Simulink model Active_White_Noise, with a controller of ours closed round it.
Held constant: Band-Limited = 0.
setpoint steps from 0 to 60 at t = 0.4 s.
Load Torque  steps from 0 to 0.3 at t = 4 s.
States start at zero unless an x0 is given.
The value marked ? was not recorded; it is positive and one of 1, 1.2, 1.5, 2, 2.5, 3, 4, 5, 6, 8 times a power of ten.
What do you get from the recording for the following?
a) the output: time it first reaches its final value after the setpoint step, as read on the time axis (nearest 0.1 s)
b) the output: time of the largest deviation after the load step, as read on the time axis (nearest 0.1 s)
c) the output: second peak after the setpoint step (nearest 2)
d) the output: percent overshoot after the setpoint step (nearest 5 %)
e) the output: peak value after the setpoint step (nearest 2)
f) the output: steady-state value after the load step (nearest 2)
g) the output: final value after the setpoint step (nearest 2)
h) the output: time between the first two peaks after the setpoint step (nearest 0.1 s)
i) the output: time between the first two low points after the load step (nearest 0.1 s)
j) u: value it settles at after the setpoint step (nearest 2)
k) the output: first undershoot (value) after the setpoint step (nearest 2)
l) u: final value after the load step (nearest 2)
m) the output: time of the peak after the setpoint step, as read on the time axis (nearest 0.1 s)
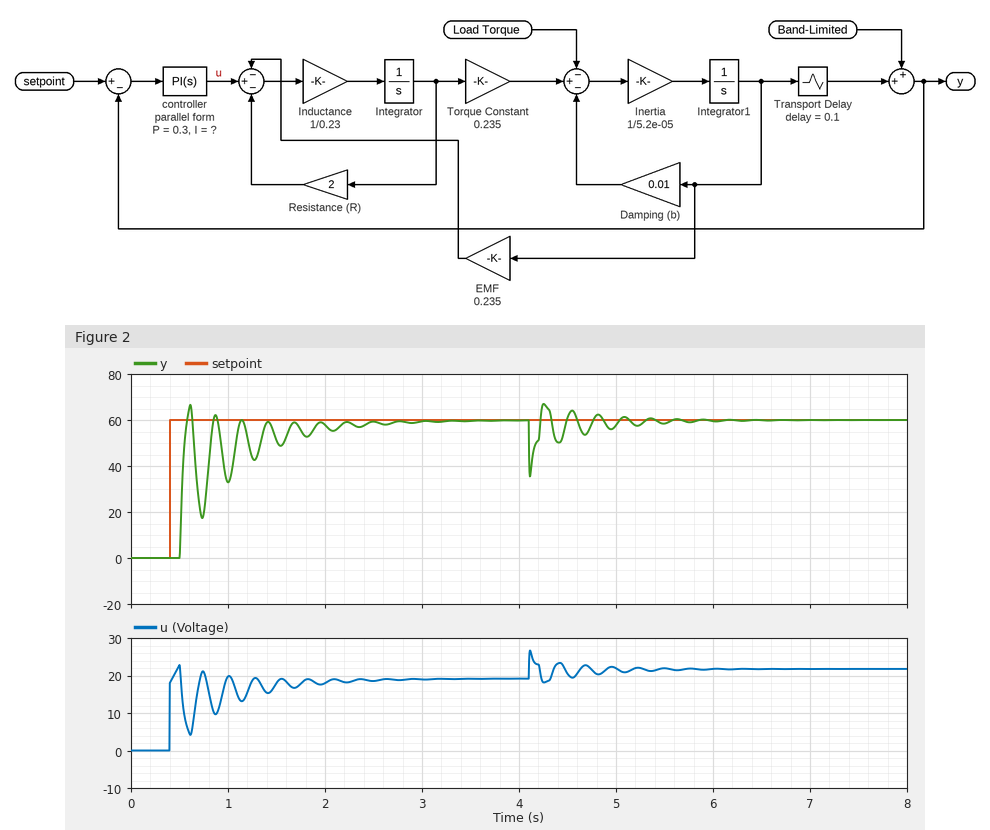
0.6 s
4.1 s
62
10 %
66
60
60
0.3 s
0.3 s
20
18
22
0.6 s
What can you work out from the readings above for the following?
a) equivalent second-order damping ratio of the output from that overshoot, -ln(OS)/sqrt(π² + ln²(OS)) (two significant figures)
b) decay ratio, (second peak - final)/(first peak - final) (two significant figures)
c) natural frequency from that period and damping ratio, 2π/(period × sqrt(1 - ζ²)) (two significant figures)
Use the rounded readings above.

0.59
0.33
26 rad/s
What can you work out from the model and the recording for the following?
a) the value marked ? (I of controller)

0.8
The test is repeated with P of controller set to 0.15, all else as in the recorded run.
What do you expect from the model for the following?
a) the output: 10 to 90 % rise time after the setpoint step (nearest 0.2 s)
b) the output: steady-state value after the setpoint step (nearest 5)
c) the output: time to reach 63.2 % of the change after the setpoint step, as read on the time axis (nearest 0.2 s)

0.8 s
60
0.6 s
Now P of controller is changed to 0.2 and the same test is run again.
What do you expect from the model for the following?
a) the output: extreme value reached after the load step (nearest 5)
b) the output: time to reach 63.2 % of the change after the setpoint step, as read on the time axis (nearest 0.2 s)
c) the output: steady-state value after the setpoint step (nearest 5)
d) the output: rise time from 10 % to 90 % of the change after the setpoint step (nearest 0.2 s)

35
0.6 s
60
1.0 s
